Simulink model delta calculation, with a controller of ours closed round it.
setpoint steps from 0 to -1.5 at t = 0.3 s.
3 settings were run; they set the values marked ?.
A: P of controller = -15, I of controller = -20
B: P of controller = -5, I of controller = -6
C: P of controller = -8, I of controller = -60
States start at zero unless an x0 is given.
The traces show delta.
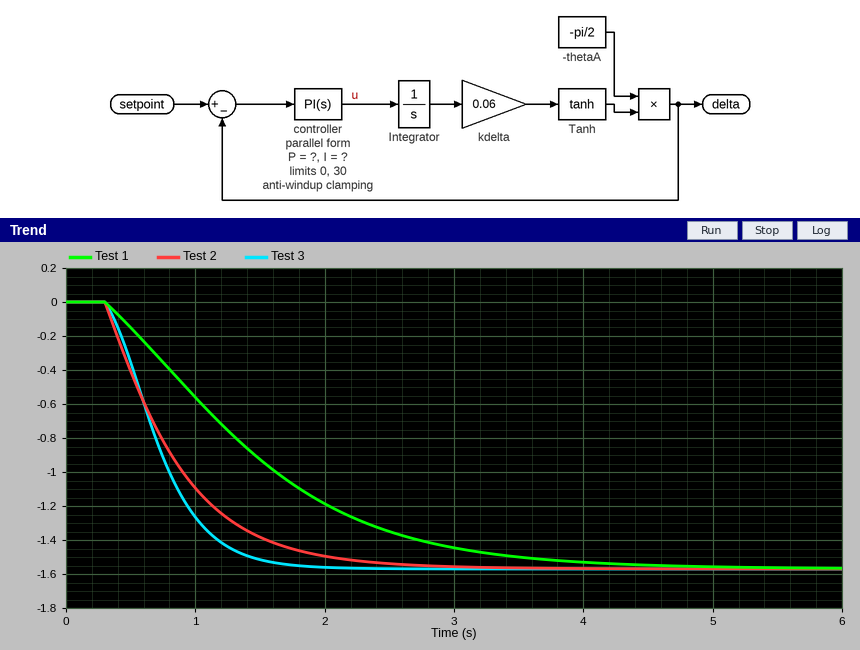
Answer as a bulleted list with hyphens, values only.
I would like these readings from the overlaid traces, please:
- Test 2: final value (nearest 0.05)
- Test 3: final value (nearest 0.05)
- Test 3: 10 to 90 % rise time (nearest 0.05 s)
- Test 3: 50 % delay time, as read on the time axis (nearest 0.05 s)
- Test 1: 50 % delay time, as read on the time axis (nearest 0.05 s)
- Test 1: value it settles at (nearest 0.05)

- -1.55
- -1.55
- 0.80 s
- 0.70 s
- 1.30 s
- -1.55
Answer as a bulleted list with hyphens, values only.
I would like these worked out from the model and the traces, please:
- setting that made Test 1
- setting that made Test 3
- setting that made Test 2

- B
- C
- A
